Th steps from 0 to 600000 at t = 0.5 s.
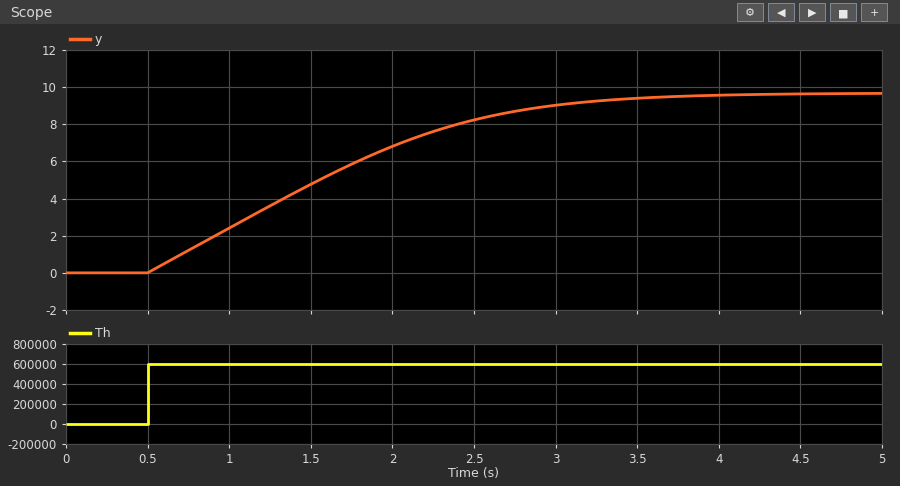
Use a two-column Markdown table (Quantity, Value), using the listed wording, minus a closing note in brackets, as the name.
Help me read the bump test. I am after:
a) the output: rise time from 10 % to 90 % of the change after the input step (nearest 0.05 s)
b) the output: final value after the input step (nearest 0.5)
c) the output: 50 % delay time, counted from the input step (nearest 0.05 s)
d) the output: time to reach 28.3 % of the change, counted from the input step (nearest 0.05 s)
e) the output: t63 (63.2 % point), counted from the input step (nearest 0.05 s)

| Quantity | Value |
|---|---|
| the output: rise time from 10 % to 90 % of the change after the input step | 2.05 s |
| the output: final value after the input step | 9.5 |
| the output: 50 % delay time, counted from the input step | 1.00 s |
| the output: time to reach 28.3 % of the change, counted from the input step | 0.55 s |
| the output: t63 (63.2 % point), counted from the input step | 1.30 s |
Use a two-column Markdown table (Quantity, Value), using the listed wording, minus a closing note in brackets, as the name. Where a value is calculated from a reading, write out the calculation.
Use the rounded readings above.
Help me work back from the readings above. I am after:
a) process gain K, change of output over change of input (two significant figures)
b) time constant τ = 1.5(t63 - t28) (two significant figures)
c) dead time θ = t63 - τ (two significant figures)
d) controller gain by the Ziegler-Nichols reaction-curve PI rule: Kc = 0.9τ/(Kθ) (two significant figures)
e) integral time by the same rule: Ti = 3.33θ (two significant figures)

| Quantity | Value |
|---|---|
| process gain K, change of output over change of input | (9.5 - 0) / 600000 = 0.000016 |
| time constant τ = 1.5(t63 - t28) | 1.5 × (1.3 - 0.55) = 1.1 s |
| dead time θ = t63 - τ | 1.3 - 1.1 = 0.20 s |
| controller gain by the Ziegler-Nichols reaction-curve PI rule: Kc = 0.9τ/(Kθ) | 0.9 × 1.1 / (1.6e-05 × 0.2) = 310000 |
| integral time by the same rule: Ti = 3.33θ | 3.33 × 0.2 = 0.67 s |
